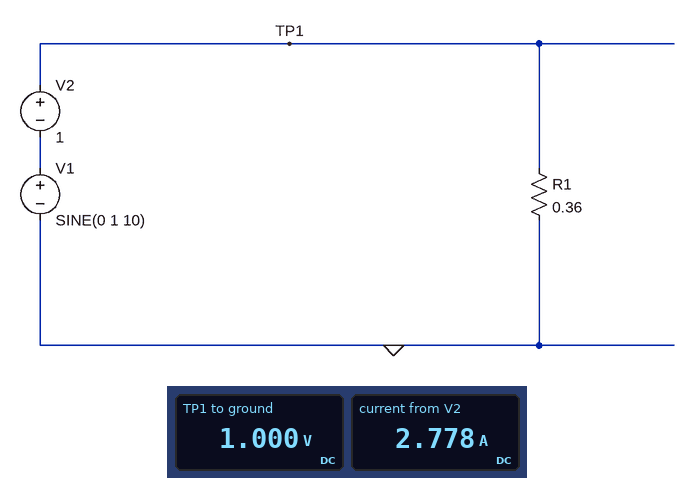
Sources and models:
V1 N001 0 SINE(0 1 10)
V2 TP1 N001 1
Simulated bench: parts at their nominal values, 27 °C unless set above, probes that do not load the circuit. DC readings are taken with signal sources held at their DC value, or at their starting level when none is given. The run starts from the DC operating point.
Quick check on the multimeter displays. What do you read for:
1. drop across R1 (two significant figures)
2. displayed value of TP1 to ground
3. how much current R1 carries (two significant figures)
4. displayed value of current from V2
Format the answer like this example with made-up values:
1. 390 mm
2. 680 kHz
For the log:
1. 1.0 V
2. 1.000 V
3. 2.8 A
4. 2.778 A
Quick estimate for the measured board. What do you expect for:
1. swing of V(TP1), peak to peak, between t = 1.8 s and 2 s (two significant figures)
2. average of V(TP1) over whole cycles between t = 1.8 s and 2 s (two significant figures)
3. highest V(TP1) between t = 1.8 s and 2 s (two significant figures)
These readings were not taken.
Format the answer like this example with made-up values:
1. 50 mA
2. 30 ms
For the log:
1. 2.0 V
2. 1.0 V
3. 2.0 V
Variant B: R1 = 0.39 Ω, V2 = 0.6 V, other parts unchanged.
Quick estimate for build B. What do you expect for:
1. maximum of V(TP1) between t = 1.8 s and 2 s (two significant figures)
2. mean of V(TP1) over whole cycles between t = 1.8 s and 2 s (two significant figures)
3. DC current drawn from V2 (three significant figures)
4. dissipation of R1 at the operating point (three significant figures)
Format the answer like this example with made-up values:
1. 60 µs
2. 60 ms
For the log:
1. 1.6 V
2. 600 mV
3. 1.54 A
4. 923 mW
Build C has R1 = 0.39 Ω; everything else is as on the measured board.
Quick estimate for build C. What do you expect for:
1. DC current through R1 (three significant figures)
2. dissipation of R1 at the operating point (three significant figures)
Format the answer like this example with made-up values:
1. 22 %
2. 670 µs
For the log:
1. 2.56 A
2. 2.56 W
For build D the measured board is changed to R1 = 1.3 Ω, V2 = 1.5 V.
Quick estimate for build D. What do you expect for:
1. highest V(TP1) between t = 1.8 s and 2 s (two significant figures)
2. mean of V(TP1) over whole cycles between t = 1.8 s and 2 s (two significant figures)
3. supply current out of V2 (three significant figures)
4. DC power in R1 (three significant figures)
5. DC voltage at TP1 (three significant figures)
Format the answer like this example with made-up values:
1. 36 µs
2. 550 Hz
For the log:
1. 2.5 V
2. 1.5 V
3. 1.15 A
4. 1.73 W
5. 1.50 V
